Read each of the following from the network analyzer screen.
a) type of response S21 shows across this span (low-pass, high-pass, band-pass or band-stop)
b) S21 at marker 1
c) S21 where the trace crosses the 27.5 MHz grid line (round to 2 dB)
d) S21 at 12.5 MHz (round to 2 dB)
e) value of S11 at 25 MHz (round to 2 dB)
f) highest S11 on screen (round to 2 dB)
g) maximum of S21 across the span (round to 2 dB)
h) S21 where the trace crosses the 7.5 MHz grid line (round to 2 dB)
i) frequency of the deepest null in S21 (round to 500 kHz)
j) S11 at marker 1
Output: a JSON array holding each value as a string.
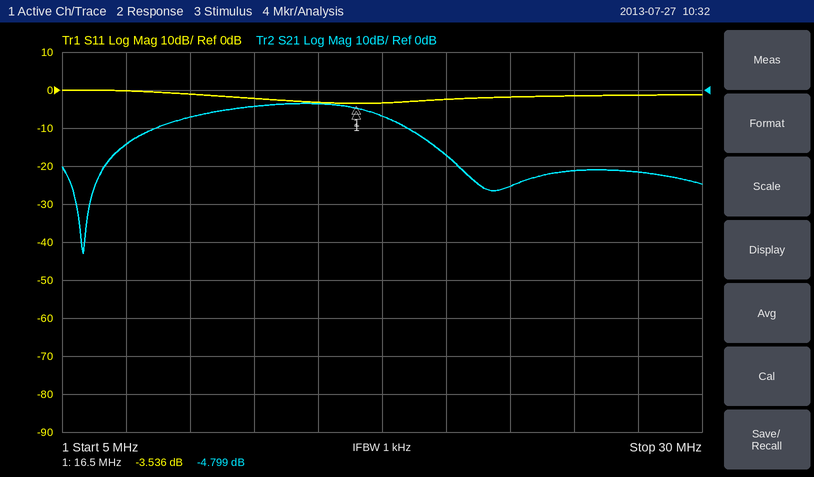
["band-pass", "-4.799 dB", "-22 dB", "-4 dB", "-2 dB", "0 dB", "-4 dB", "-14 dB", "6.0 MHz", "-3.536 dB"]
